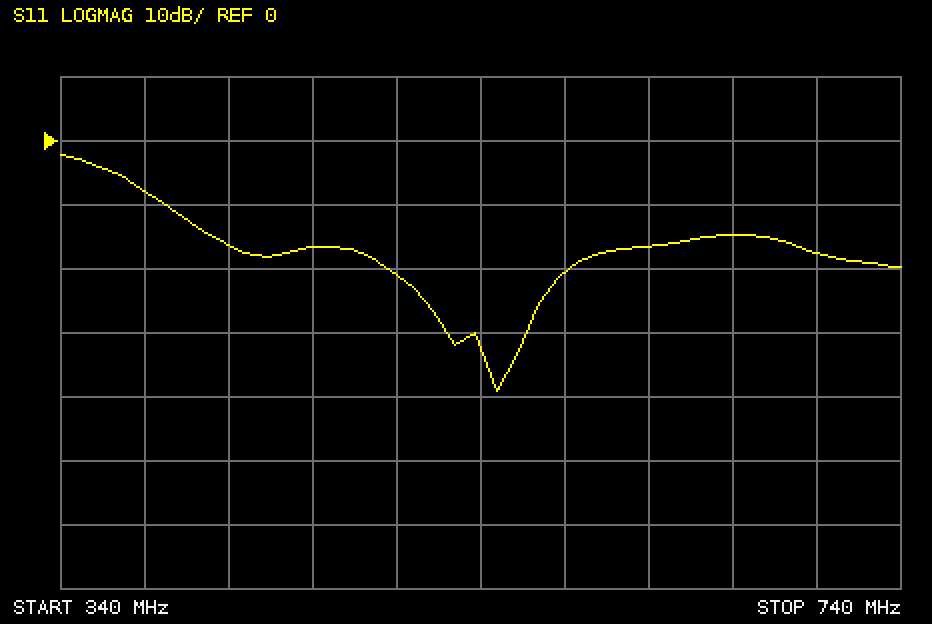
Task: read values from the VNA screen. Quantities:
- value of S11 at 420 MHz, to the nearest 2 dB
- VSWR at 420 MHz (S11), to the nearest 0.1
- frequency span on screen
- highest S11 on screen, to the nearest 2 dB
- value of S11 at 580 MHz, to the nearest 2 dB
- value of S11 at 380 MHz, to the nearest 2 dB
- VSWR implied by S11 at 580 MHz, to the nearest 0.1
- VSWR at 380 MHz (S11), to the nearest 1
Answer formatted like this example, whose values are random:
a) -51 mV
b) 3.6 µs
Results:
a) -16 dB
b) 1.4
c) 400 MHz
d) -2 dB
e) -20 dB
f) -8 dB
g) 1.2
h) 2
